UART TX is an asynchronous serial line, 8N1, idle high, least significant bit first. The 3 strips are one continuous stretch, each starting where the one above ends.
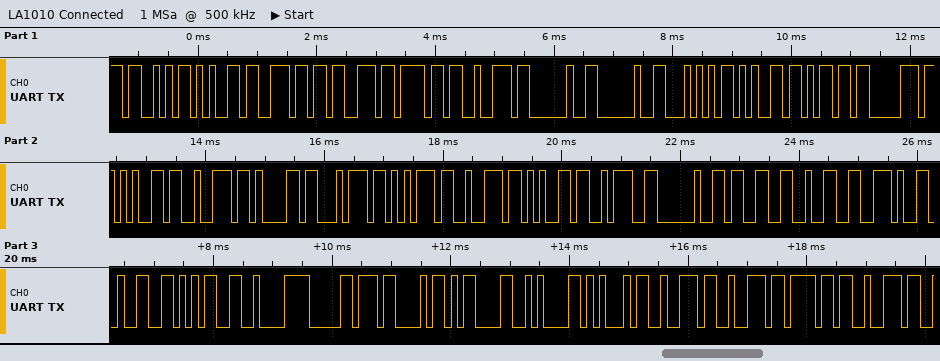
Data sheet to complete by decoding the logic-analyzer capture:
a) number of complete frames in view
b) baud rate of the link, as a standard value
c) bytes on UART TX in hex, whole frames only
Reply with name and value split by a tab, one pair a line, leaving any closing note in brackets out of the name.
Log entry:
number of complete frames in view	36
baud rate of the link, as a standard value	9600 baud
bytes on UART TX in hex, whole frames only	0x53 0x65 0x6E 0x73 0x6F 0x72 0x20 0x20 0x54 0x65 0x6D 0x70 0x65 0x72 0x61 0x74 0x75 0x72 0x65 0x3A 0x20 0x33 0x32 0x2E 0x32 0x35 0xC2 0xB0 0x43 0x0D 0x0A 0x45 0x72 0x72 0x6F 0x72
